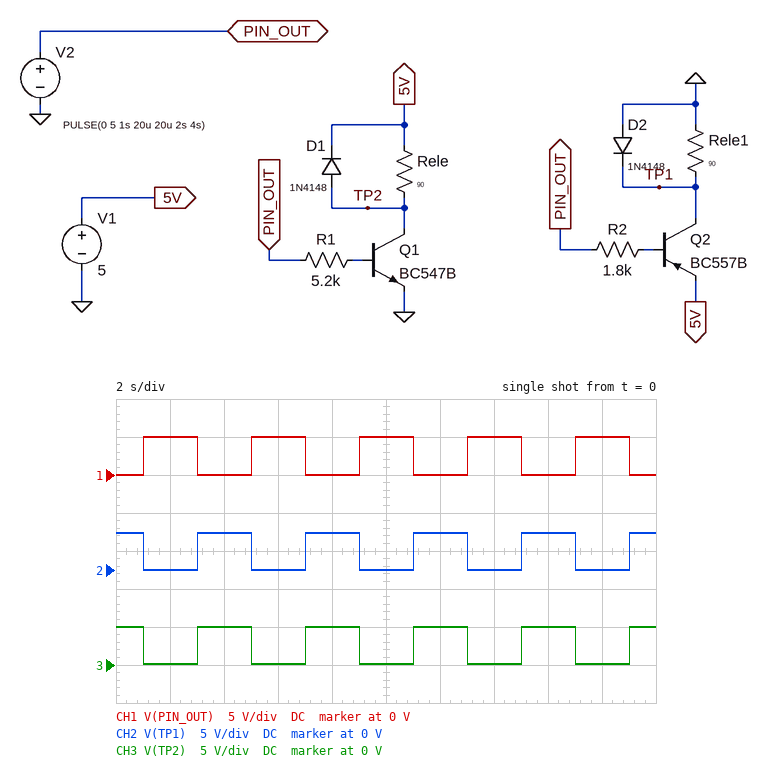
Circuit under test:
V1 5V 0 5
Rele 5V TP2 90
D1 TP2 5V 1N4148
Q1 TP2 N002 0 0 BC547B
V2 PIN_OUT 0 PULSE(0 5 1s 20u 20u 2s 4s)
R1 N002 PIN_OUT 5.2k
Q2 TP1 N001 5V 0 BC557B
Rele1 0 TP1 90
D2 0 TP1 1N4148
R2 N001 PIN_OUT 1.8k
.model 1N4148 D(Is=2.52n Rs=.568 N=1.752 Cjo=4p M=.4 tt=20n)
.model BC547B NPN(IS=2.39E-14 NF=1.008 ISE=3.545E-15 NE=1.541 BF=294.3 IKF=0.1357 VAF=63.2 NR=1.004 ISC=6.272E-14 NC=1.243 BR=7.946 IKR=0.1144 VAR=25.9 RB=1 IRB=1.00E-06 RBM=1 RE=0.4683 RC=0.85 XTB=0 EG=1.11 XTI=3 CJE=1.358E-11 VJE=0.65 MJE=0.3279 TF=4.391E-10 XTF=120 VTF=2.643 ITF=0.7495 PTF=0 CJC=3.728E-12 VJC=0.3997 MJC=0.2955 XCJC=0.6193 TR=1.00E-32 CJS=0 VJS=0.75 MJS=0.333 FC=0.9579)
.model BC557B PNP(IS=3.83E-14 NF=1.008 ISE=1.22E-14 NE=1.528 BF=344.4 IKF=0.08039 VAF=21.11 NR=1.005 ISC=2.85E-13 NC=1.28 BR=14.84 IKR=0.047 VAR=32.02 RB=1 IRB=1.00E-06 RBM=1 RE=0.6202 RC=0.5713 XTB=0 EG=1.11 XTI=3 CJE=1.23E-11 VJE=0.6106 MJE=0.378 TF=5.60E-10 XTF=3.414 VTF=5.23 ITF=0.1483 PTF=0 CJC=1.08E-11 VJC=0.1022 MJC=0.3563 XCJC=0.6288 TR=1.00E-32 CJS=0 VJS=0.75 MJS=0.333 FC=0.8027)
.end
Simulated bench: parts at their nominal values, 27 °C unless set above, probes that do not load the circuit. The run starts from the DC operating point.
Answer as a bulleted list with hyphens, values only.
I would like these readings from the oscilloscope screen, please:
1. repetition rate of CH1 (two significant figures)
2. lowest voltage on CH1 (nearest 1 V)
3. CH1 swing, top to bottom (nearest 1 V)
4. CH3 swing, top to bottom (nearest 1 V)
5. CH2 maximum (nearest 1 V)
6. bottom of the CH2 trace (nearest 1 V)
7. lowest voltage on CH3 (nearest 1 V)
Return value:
- 250 mHz
- 0 V
- 5 V
- 5 V
- 5 V
- 0 V
- 0 V
